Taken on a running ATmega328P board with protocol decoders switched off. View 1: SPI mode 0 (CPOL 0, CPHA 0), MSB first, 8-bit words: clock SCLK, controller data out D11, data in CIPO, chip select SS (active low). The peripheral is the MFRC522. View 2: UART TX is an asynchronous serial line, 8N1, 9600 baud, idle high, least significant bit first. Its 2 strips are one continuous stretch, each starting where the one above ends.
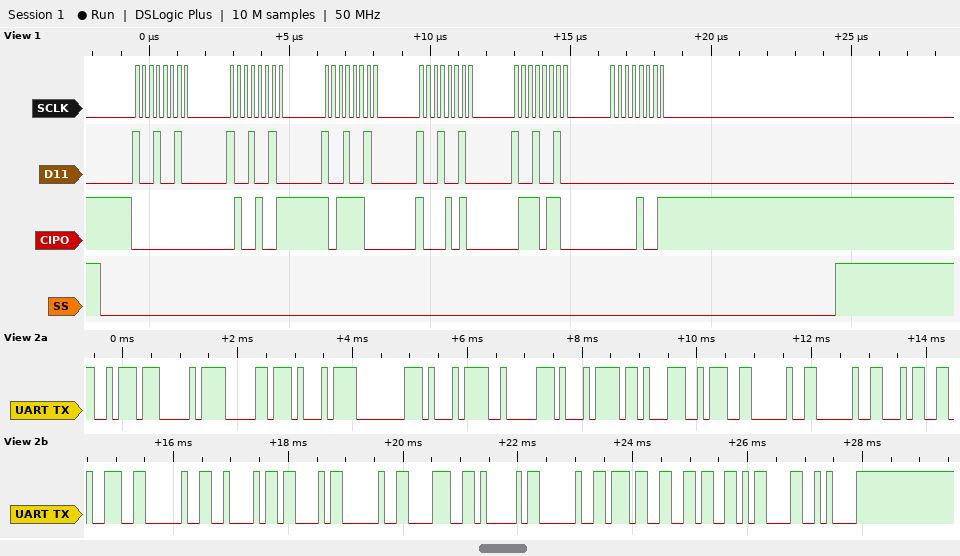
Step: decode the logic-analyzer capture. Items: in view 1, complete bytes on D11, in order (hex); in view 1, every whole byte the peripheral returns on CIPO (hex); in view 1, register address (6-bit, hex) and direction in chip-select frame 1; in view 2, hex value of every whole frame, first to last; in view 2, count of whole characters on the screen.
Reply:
0x92 0x92 0x92 0x92 0x92 0x00
0x00 0x49 0xBC 0x8A 0x76 0x09
0x09 read
BA D0 B0 D1 80 D1 82 D1 8B 3A 20 20 34 39 20 42 43 20 38 41 20 37 36 0D 0A
25
